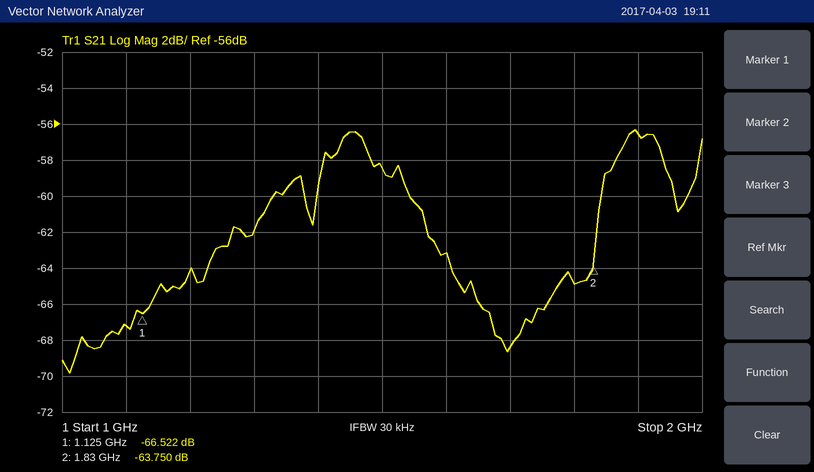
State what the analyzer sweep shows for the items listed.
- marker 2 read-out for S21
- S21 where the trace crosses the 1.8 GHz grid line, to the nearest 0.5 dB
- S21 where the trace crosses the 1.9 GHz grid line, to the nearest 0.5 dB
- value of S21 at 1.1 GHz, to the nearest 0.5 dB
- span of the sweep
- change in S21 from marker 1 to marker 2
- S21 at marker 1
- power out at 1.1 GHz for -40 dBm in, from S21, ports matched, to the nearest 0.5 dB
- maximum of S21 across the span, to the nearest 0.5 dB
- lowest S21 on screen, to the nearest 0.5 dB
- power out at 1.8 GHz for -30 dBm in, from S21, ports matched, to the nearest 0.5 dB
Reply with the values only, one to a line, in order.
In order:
-63.750 dB
-65.0 dB
-56.5 dB
-67.0 dB
1 GHz
2.772 dB
-66.522 dB
-107.0 dBm
-56.5 dB
-70.0 dB
-95.0 dBm
